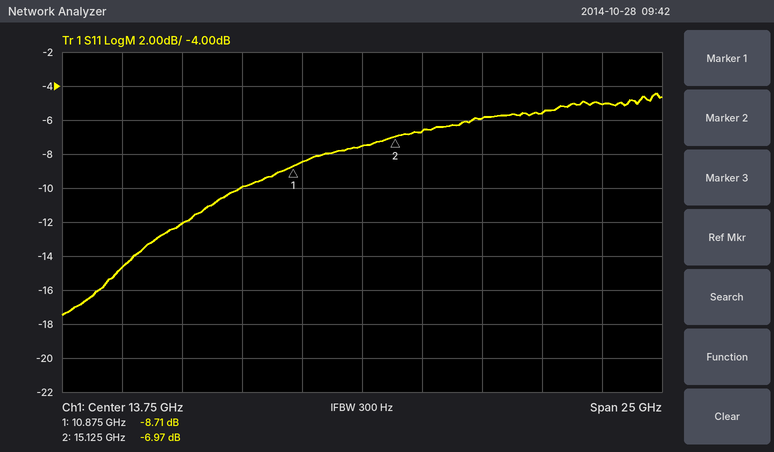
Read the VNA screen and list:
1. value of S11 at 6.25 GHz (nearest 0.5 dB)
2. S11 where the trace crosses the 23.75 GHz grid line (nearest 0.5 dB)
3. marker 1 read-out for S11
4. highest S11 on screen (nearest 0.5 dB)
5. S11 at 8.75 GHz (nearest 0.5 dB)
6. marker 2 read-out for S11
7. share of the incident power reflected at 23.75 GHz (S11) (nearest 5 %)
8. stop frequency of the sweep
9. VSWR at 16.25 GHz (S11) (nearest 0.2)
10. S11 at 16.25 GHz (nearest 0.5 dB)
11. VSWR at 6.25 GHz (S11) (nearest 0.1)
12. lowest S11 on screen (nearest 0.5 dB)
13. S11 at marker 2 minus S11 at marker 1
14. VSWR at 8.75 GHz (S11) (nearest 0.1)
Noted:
-12.0 dB
-5.0 dB
-8.71 dB
-4.5 dB
-10.0 dB
-6.97 dB
30 %
26.25 GHz
2.8
-6.5 dB
1.7
-17.5 dB
1.74 dB
1.9
